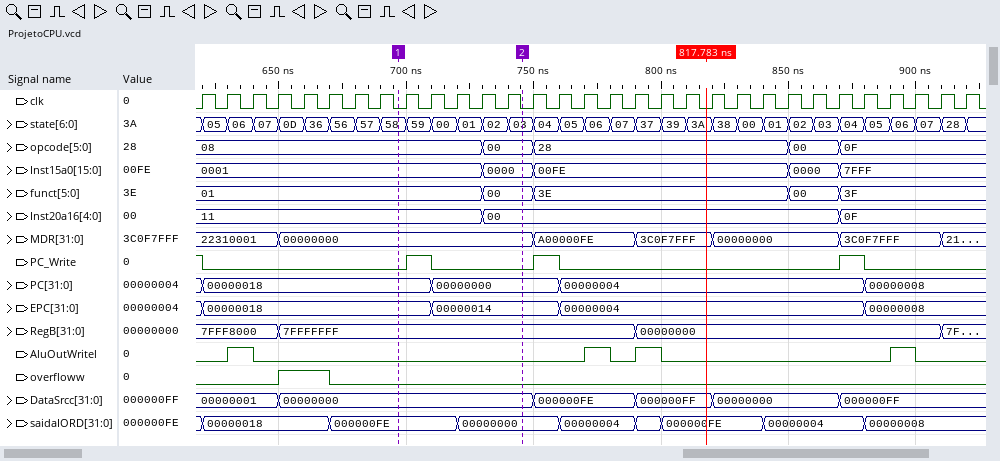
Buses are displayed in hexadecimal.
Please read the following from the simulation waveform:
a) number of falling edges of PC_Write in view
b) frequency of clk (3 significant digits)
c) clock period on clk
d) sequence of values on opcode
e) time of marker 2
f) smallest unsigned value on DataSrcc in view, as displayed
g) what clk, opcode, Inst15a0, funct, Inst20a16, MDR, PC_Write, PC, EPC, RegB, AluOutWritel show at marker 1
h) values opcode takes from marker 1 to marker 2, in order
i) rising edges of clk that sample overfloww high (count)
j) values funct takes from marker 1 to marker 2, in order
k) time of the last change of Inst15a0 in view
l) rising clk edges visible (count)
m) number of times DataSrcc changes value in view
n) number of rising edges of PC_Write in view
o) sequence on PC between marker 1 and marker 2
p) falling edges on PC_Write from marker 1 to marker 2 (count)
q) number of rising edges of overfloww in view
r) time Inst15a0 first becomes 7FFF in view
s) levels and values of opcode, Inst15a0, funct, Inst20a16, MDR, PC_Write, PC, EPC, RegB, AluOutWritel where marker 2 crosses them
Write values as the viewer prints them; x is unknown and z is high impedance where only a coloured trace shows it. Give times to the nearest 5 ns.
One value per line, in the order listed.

4
100 MHz
10 ns
08, 00, 28, 00, 0F
745 ns
00000000
clk=0, opcode=08, Inst15a0=0001, funct=01, Inst20a16=11, MDR=00000000, PC_Write=0, PC=00000018, EPC=00000018, RegB=7FFFFFFF, AluOutWritel=0
08, 00
2
01, 00
870 ns
31
5
3
00000018, 00000000
1
1
870 ns
opcode=00, Inst15a0=0000, funct=00, Inst20a16=00, MDR=00000000, PC_Write=0, PC=00000000, EPC=00000014, RegB=7FFFFFFF, AluOutWritel=0
